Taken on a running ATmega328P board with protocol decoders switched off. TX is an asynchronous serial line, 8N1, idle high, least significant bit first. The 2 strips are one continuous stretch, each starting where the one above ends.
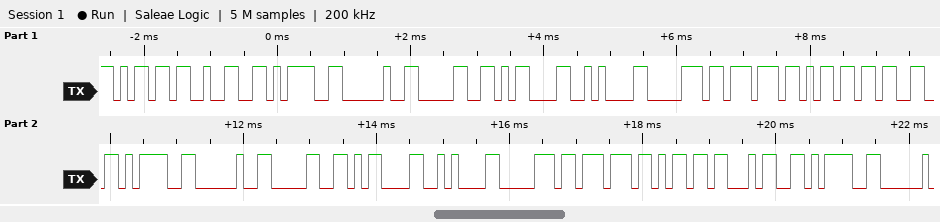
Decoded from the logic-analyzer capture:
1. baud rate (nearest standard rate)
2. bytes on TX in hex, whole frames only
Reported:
9600 baud
0x6D 0x32 0x3D 0x20 0x30 0x0D 0x0A 0x70 0x77 0x6D 0x33 0x3D 0x20 0x30 0x0D 0x0A 0x70 0x77 0x6D 0x34 0x3D
